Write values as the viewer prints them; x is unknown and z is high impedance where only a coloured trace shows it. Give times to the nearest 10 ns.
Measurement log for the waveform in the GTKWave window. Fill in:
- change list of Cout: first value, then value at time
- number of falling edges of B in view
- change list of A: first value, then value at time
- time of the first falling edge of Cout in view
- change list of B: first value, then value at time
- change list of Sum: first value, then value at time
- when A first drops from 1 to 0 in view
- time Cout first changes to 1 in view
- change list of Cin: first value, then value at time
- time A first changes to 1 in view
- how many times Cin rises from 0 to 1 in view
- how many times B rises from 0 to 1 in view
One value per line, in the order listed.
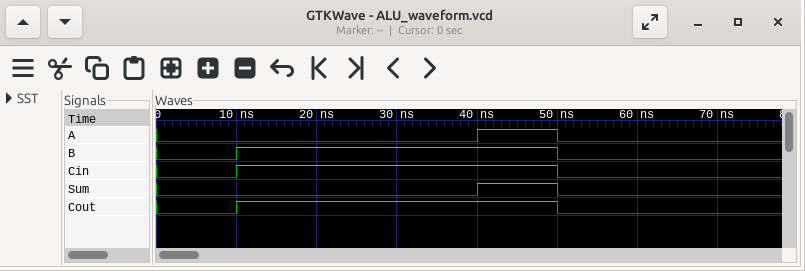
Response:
0, 1 at 10 ns, 0 at 50 ns
1
0, 1 at 40 ns, 0 at 50 ns
50 ns
0, 1 at 10 ns, 0 at 50 ns
0, 1 at 40 ns, 0 at 50 ns
50 ns
10 ns
0, 1 at 10 ns, 0 at 50 ns
40 ns
1
1
